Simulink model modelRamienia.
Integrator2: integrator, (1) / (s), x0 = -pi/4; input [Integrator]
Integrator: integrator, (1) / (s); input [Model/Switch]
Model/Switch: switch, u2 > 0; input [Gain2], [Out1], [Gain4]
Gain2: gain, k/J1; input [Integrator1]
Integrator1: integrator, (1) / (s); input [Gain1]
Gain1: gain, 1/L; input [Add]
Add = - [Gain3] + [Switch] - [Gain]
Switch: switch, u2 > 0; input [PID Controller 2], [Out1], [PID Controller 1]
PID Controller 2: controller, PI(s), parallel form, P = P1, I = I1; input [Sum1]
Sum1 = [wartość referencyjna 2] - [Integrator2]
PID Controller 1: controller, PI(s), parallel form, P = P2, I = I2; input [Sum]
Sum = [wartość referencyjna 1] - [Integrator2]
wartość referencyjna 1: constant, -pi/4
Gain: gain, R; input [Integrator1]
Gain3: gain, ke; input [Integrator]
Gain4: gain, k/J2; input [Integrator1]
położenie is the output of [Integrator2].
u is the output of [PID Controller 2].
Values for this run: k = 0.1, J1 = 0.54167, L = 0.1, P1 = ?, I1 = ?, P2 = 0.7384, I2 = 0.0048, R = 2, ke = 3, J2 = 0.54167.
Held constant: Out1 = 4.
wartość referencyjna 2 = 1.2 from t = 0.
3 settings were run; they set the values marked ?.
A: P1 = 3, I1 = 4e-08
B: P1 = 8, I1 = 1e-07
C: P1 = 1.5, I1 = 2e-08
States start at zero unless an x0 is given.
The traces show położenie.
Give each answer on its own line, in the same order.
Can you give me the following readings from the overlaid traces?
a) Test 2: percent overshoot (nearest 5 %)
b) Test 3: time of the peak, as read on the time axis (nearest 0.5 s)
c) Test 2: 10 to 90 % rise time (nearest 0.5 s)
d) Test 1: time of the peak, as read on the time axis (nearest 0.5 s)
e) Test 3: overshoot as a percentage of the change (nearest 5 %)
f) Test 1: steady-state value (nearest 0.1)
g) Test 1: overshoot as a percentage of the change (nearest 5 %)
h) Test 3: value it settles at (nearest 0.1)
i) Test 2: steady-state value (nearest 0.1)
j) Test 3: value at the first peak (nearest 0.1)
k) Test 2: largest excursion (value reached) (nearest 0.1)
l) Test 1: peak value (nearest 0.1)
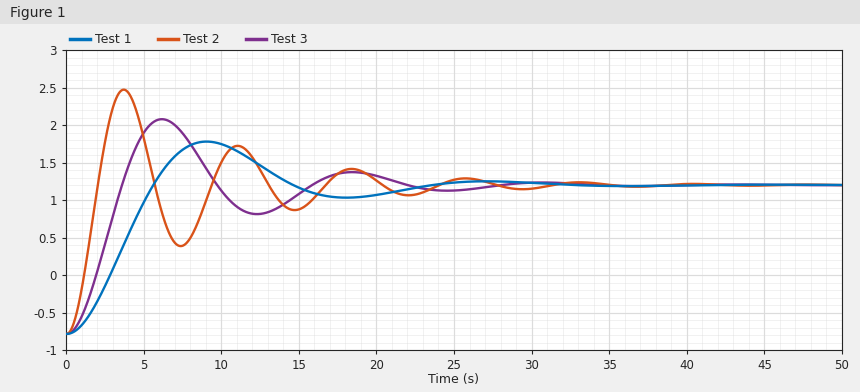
65 %
6.0 s
1.5 s
9.0 s
45 %
1.2
30 %
1.2
1.2
2.1
2.5
1.8
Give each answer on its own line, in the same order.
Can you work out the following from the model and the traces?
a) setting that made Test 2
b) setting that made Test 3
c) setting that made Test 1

B
A
C
